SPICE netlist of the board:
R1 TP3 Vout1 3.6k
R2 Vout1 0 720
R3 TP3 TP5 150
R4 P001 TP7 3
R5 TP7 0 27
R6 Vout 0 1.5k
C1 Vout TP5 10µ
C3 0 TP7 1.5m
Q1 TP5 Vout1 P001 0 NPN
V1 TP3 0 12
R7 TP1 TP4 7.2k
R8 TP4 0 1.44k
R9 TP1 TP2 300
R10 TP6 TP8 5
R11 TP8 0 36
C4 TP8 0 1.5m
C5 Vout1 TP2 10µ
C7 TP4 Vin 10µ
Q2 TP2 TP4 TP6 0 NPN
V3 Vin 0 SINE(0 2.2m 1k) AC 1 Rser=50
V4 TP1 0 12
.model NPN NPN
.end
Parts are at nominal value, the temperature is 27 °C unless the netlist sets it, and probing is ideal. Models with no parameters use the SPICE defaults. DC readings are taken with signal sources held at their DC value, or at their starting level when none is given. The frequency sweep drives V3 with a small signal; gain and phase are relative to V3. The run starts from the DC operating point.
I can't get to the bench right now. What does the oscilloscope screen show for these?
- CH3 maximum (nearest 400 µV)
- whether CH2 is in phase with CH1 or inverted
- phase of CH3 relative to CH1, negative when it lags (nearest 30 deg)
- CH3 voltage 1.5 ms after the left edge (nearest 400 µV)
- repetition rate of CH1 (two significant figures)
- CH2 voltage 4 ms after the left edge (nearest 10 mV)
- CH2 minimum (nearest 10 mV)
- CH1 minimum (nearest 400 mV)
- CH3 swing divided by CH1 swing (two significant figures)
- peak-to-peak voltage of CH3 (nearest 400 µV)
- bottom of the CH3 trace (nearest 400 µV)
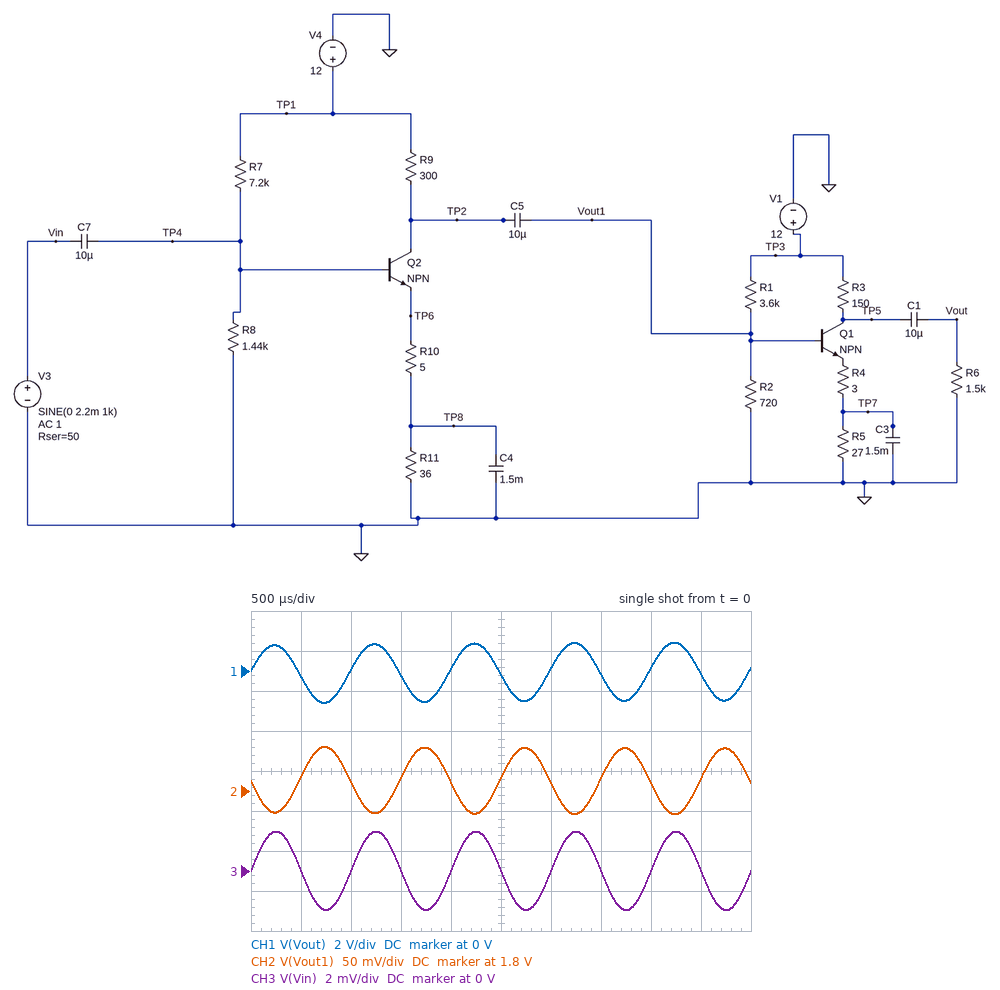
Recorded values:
2.0 mV
inverted
0 deg
0 V
1.0 kHz
1.81 V
1.77 V
-1.6 V
0.0013
4.0 mV
-2.0 mV
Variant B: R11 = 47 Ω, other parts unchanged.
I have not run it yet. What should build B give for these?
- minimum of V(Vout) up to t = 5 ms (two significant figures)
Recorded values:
-1.5 V
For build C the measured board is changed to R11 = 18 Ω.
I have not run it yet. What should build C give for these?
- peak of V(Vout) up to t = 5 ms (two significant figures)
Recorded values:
1.5 V
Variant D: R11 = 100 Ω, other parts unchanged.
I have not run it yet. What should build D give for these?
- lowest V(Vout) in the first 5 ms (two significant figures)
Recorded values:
-1.3 V
